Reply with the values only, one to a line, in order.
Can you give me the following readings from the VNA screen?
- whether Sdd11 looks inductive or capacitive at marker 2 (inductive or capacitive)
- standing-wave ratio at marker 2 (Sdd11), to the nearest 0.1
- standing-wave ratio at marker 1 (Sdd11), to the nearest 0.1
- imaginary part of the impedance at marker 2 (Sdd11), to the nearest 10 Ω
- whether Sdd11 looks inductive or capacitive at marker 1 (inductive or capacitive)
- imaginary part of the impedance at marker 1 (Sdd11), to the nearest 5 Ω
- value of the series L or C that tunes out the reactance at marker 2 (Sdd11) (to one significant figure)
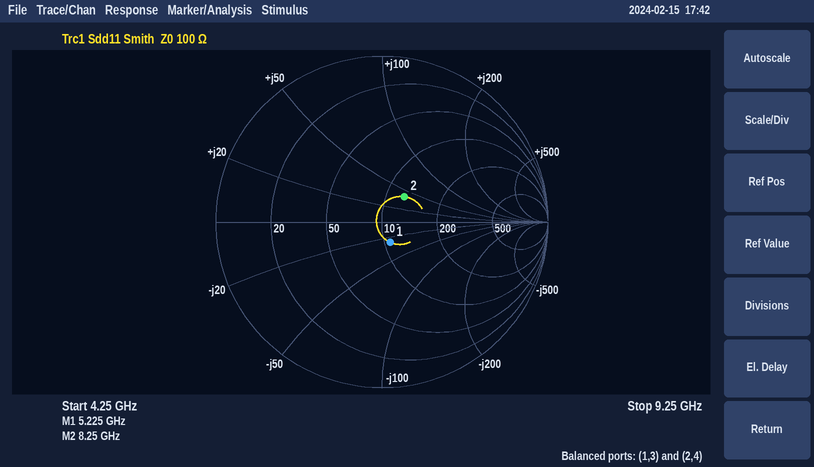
inductive
1.5
1.3
+40 Ω
capacitive
-25 Ω
500 fF
